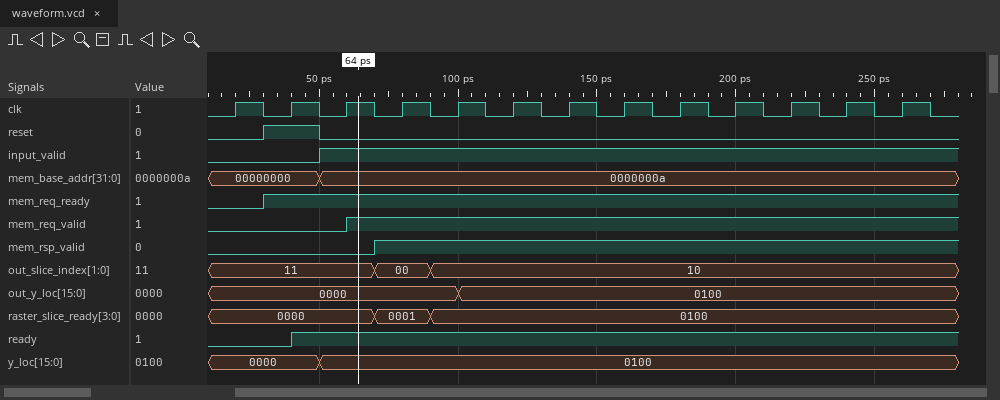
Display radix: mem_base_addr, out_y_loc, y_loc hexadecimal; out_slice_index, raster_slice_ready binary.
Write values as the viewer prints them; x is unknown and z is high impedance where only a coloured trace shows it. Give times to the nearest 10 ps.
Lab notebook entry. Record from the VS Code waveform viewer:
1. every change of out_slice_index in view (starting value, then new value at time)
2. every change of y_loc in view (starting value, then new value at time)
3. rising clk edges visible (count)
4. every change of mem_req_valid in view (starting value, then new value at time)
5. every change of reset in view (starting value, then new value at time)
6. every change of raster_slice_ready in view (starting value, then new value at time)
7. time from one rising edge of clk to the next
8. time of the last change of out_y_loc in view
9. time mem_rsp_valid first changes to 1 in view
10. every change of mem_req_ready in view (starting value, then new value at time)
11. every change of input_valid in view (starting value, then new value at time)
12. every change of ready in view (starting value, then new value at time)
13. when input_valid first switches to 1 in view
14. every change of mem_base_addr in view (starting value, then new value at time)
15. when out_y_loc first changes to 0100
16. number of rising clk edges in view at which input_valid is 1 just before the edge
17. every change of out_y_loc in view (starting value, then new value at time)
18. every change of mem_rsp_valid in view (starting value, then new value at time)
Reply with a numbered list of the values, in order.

1. 11, 00 at 70 ps, 10 at 90 ps
2. 0000, 0100 at 50 ps
3. 13
4. 0, 1 at 60 ps
5. 0, 1 at 30 ps, 0 at 50 ps
6. 0000, 0001 at 70 ps, 0100 at 90 ps
7. 20 ps
8. 100 ps
9. 70 ps
10. 0, 1 at 30 ps
11. 0, 1 at 50 ps
12. 0, 1 at 40 ps
13. 50 ps
14. 00000000, 0000000a at 50 ps
15. 100 ps
16. 11
17. 0000, 0100 at 100 ps
18. 0, 1 at 70 ps
